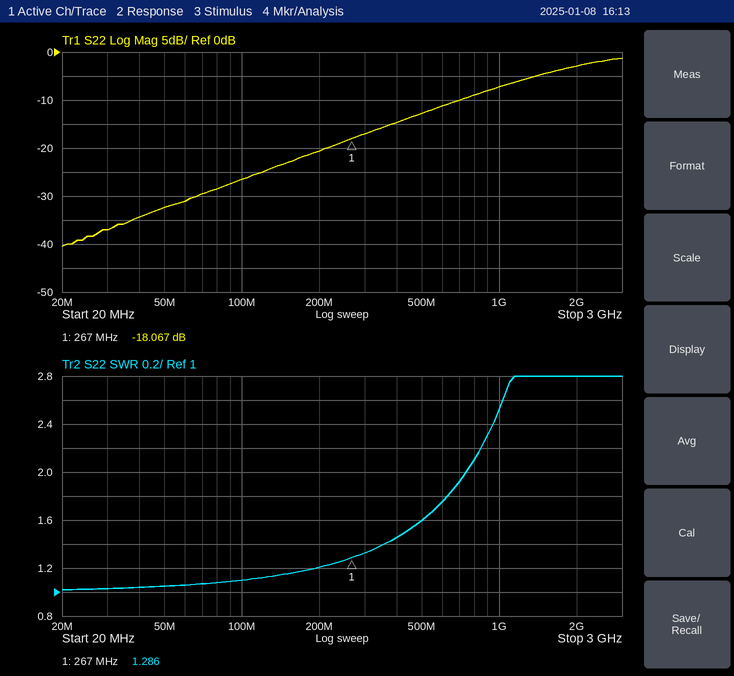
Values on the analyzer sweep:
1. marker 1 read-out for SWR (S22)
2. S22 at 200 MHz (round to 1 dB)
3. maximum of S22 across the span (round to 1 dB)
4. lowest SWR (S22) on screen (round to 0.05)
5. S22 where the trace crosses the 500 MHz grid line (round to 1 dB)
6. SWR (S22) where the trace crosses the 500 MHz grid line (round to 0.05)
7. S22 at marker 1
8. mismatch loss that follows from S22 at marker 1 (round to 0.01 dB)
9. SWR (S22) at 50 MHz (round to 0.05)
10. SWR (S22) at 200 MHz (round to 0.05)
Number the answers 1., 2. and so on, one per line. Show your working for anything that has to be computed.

1. 1.286
2. -21 dB
3. -1 dB
4. 1.00
5. -13 dB
6. 1.60
7. -18.067 dB
8. −10 log10(1 − 10^(-18.067/10)) ≈ 0.07 dB
9. 1.05
10. 1.20
